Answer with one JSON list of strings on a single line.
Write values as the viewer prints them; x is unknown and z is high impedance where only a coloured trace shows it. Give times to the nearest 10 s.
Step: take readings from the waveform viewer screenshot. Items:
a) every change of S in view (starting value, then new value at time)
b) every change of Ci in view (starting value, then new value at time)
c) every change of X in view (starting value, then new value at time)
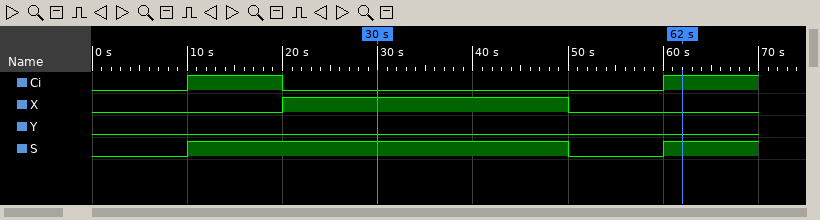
["0, 1 at 10 s, 0 at 50 s, 1 at 60 s", "0, 1 at 10 s, 0 at 20 s, 1 at 60 s", "0, 1 at 20 s, 0 at 50 s"]
